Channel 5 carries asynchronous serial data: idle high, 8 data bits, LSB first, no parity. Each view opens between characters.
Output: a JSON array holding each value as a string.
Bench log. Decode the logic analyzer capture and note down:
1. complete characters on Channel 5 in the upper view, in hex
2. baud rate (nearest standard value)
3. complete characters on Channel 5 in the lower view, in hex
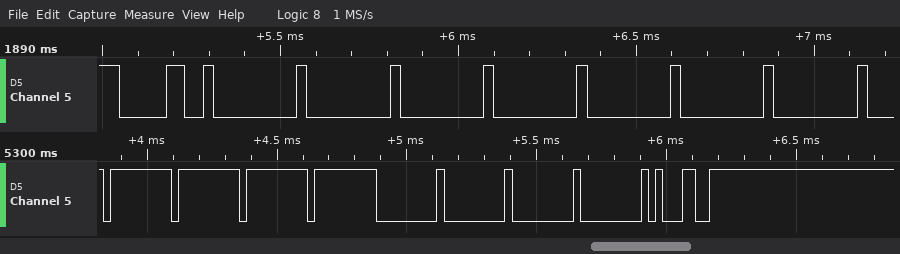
["30, 00, 00, 00, 00, 00, 00, 00", "38400 baud", "FF, FF, FF, FF, 00, 00, 00, 00, 31"]
